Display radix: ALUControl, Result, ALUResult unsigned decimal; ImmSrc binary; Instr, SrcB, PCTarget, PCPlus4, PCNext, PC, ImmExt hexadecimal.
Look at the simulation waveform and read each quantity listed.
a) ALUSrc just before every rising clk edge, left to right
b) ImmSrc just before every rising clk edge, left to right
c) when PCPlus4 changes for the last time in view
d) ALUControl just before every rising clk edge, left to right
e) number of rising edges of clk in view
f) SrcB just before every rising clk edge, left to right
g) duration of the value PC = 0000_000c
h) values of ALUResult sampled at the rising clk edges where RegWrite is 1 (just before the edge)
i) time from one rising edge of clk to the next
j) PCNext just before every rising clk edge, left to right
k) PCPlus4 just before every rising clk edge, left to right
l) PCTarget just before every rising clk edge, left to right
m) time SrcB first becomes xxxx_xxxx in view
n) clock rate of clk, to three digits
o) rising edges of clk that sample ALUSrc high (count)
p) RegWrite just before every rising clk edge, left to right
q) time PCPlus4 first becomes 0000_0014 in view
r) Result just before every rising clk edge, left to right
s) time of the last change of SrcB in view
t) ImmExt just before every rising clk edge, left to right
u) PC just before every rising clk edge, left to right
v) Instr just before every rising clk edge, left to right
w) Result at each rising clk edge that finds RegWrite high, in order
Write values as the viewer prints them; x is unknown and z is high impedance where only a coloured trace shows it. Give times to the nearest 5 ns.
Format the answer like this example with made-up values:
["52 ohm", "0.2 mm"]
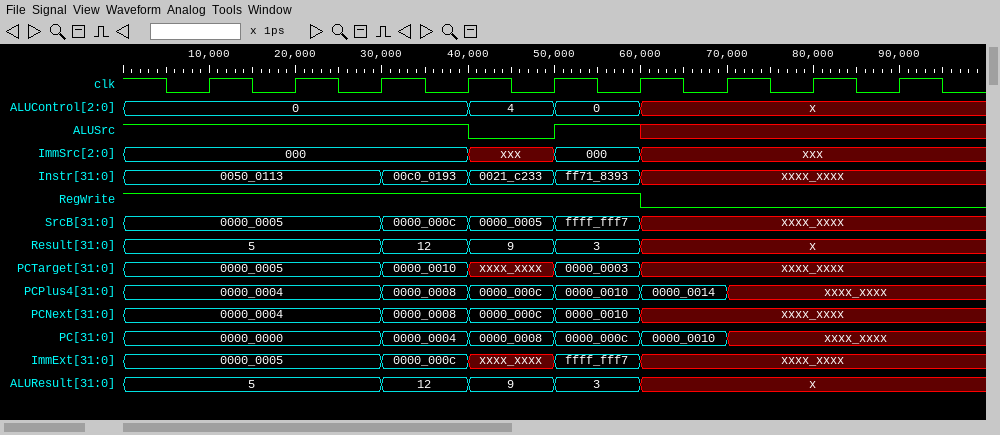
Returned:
["1 1 1 1 0 1 x x x", "000, 000, 000, 000, xxx, 000, xxx, xxx, xxx", "70 ns", "0, 0, 0, 0, 4, 0, x, x, x", "9", "0000_0005, 0000_0005, 0000_0005, 0000_000c, 0000_0005, ffff_fff7, xxxx_xxxx, xxxx_xxxx, xxxx_xxxx", "10 ns", "5, 5, 5, 12, 9, 3", "10 ns", "0000_0004, 0000_0004, 0000_0004, 0000_0008, 0000_000c, 0000_0010, xxxx_xxxx, xxxx_xxxx, xxxx_xxxx", "0000_0004, 0000_0004, 0000_0004, 0000_0008, 0000_000c, 0000_0010, 0000_0014, xxxx_xxxx, xxxx_xxxx", "0000_0005, 0000_0005, 0000_0005, 0000_0010, xxxx_xxxx, 0000_0003, xxxx_xxxx, xxxx_xxxx, xxxx_xxxx", "60 ns", "100 MHz", "5", "1 1 1 1 1 1 0 0 0", "60 ns", "5, 5, 5, 12, 9, 3, x, x, x", "60 ns", "0000_0005, 0000_0005, 0000_0005, 0000_000c, xxxx_xxxx, ffff_fff7, xxxx_xxxx, xxxx_xxxx, xxxx_xxxx", "0000_0000, 0000_0000, 0000_0000, 0000_0004, 0000_0008, 0000_000c, 0000_0010, xxxx_xxxx, xxxx_xxxx", "0050_0113, 0050_0113, 0050_0113, 00c0_0193, 0021_c233, ff71_8393, xxxx_xxxx, xxxx_xxxx, xxxx_xxxx", "5, 5, 5, 12, 9, 3"]
